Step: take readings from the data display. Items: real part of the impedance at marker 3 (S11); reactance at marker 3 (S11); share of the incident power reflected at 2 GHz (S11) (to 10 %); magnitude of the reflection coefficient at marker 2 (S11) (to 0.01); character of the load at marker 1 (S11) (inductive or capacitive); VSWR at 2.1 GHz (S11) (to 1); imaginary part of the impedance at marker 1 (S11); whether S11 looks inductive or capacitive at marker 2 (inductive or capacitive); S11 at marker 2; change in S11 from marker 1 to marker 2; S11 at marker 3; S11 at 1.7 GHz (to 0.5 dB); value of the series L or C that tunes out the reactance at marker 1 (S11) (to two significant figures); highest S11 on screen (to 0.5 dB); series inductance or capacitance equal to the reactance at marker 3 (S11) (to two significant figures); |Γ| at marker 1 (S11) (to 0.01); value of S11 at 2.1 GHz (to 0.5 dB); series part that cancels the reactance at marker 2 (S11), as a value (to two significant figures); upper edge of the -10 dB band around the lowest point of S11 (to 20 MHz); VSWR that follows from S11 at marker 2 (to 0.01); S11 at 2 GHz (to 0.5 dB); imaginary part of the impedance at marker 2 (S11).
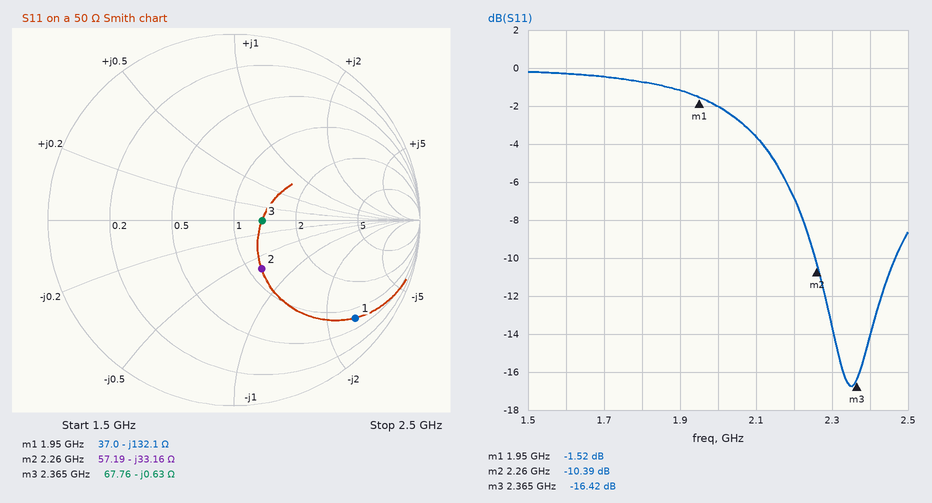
67.76 Ω
-0.63 Ω
60 %
0.30
capacitive
5
-132.1 Ω
capacitive
-10.39 dB
-8.87 dB
-16.42 dB
-0.5 dB
11 nH
0.0 dB
110 pF
0.84
-3.5 dB
2.3 nH
2.46 GHz
1.87
-2.0 dB
-33.16 Ω
